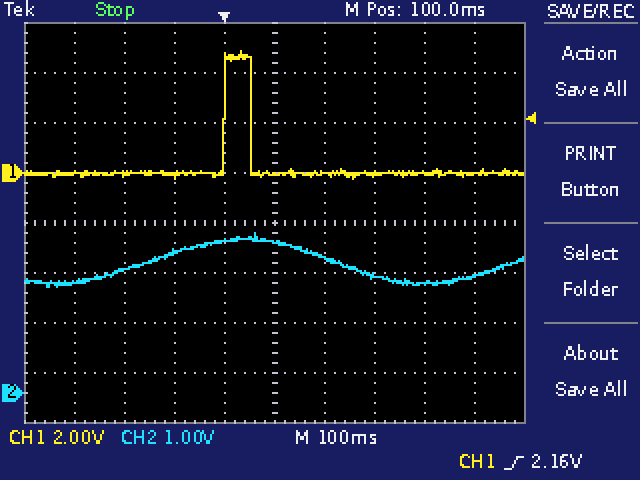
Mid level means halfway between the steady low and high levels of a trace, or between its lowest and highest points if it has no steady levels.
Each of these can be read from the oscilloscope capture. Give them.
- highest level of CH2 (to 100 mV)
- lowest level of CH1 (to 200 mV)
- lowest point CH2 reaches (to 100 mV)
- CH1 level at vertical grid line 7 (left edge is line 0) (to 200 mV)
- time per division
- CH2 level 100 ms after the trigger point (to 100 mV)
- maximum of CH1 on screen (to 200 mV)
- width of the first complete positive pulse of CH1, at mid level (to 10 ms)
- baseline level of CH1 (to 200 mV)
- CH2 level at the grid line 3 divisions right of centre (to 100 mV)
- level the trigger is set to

3.2 V
-200 mV
2.1 V
0.0 V
100 ms
3.0 V
4.8 V
50 ms
0.0 V
2.2 V
2.16 V
